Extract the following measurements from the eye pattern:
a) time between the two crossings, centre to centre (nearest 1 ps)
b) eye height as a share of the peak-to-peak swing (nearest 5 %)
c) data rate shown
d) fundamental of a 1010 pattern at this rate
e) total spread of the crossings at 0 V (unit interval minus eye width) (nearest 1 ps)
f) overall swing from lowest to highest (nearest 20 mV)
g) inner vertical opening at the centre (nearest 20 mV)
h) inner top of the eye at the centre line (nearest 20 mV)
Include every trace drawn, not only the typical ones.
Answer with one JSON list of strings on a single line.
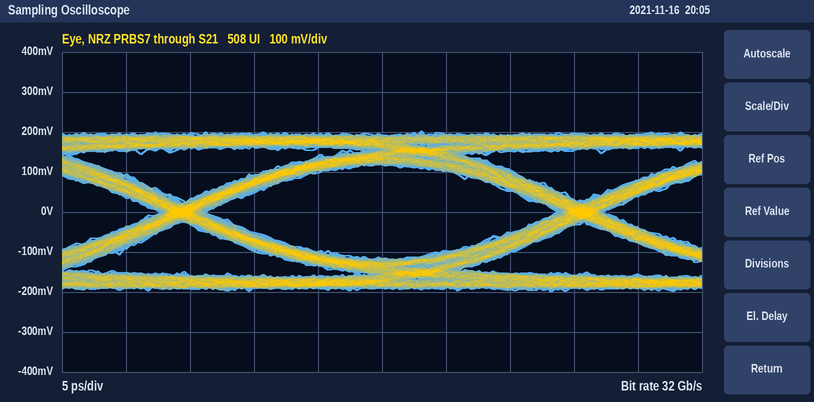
["31 ps", "60 %", "32 Gb/s", "16 GHz", "4 ps", "400 mV", "240 mV", "120 mV"]
